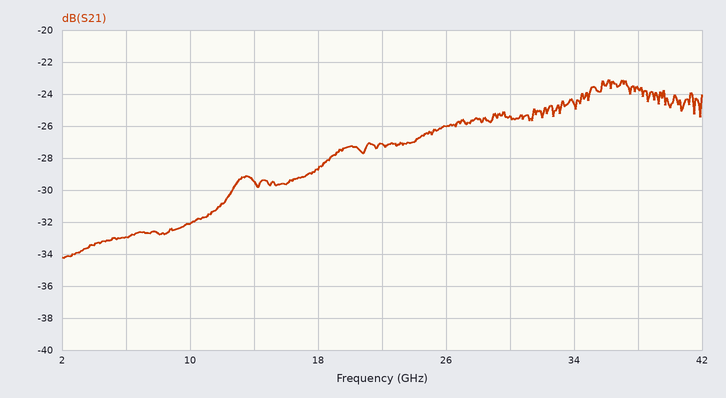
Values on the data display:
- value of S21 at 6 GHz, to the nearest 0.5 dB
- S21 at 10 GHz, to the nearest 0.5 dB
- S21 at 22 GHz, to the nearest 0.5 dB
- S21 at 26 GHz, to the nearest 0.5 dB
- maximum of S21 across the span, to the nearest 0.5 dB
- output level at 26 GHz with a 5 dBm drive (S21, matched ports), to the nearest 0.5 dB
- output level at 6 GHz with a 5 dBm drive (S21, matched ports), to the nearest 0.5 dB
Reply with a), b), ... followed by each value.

a) -33.0 dB
b) -32.0 dB
c) -27.0 dB
d) -26.0 dB
e) -23.0 dB
f) -21.0 dBm
g) -28.0 dBm
